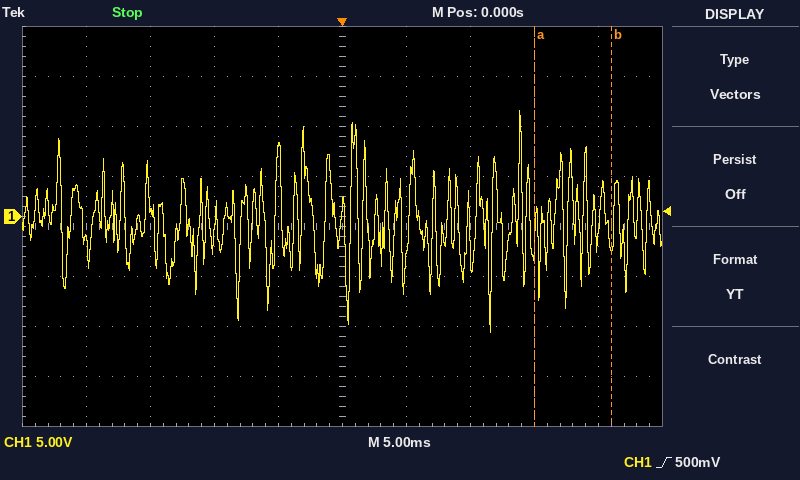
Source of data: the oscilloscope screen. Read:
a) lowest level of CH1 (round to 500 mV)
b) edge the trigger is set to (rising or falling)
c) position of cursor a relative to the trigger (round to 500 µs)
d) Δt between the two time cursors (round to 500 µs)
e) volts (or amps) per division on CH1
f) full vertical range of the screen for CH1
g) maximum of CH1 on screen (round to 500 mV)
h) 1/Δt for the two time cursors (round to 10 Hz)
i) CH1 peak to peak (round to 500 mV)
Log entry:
-11.5 V
rising
+15.0 ms
6.0 ms
5 V
40 V
10.5 V
170 Hz
22.0 V
